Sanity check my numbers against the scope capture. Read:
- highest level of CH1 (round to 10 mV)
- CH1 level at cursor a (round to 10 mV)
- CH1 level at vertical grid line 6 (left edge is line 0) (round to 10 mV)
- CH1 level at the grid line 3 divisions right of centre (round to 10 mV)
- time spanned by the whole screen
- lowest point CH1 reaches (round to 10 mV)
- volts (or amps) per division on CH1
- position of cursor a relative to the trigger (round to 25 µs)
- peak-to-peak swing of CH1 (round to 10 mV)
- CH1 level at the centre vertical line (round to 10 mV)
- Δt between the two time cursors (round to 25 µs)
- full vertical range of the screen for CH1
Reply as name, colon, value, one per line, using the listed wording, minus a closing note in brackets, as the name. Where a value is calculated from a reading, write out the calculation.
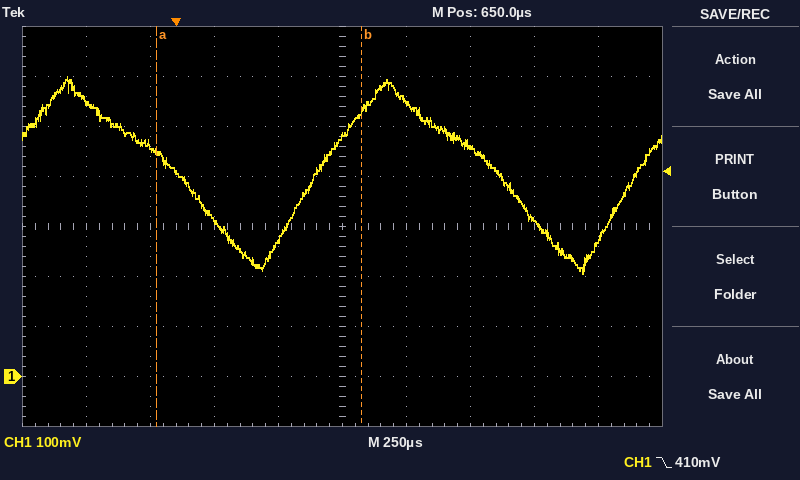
highest level of CH1: 600 mV
CH1 level at cursor a: 450 mV
CH1 level at vertical grid line 6 (left edge is line 0): 550 mV
CH1 level at the grid line 3 divisions right of centre: 310 mV
time spanned by the whole screen: 2.5 ms
lowest point CH1 reaches: 210 mV
volts (or amps) per division on CH1: 100 mV
position of cursor a relative to the trigger: -75 µs
peak-to-peak swing of CH1: 600 mV − (210 mV) = 390 mV
CH1 level at the centre vertical line: 480 mV
Δt between the two time cursors: 800 µs
full vertical range of the screen for CH1: 800 mV
